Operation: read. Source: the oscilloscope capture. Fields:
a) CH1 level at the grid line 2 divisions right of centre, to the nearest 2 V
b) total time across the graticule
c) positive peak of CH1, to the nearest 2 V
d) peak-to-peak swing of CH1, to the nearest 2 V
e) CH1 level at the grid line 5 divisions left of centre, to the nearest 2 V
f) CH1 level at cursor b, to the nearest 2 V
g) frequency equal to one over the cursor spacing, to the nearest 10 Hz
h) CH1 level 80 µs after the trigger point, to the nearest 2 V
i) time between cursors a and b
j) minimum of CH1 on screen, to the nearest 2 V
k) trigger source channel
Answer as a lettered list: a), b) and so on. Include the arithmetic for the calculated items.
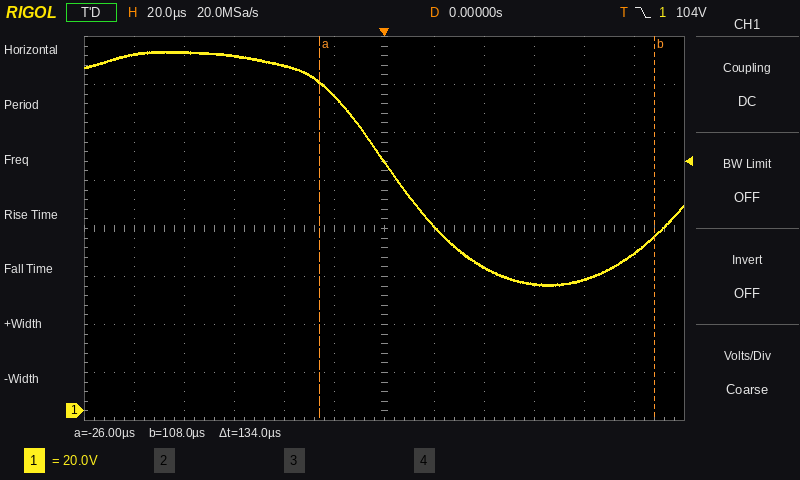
a) 60 V
b) 240 µs
c) 150 V
d) 150 V − (52 V) = 98 V
e) 148 V
f) 72 V
g) 1 / 134 µs ≈ 7.46 kHz
h) 54 V
i) 134 µs
j) 52 V
k) CH1
